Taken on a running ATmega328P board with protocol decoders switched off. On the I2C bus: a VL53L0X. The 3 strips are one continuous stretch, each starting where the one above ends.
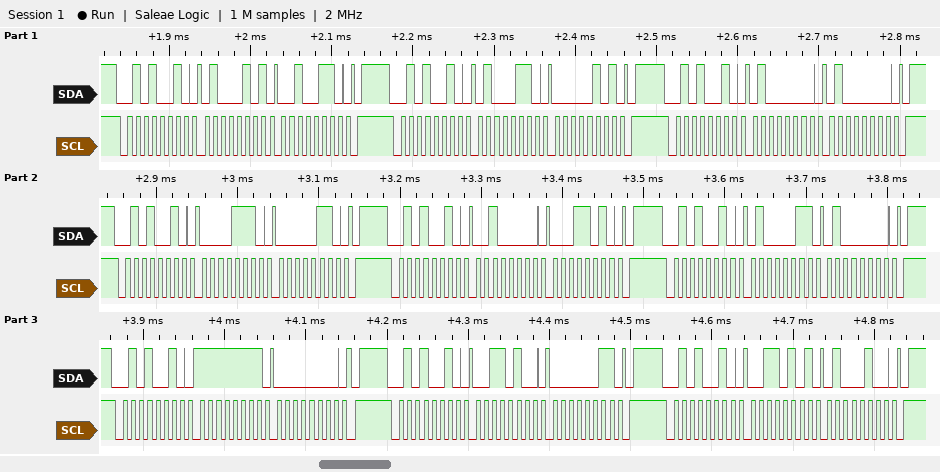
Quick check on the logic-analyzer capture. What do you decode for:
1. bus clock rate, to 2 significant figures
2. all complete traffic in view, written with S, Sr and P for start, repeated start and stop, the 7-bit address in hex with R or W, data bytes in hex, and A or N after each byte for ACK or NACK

100 kHz
S 29W A 45 A 26 A P S 29W A 46 A 05 A P S 29W A 40 A 40 A P S 29W A 0E A 06 A P S 29W A 20 A 1A A P S 29W A 43 A 40 A P S 29W A FF A 00 A P S 29W A 34 A 03 A P S 29W A 35 A 44 A P
